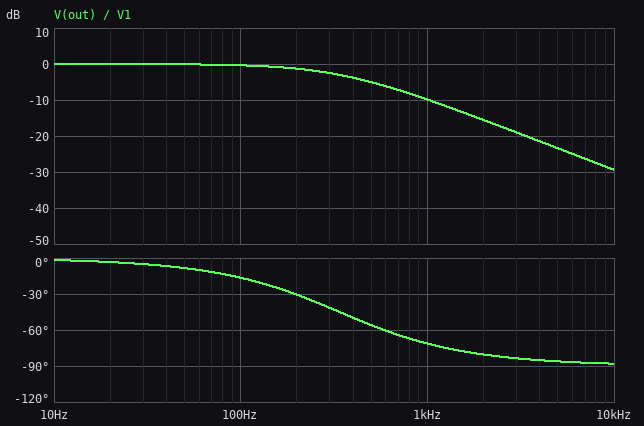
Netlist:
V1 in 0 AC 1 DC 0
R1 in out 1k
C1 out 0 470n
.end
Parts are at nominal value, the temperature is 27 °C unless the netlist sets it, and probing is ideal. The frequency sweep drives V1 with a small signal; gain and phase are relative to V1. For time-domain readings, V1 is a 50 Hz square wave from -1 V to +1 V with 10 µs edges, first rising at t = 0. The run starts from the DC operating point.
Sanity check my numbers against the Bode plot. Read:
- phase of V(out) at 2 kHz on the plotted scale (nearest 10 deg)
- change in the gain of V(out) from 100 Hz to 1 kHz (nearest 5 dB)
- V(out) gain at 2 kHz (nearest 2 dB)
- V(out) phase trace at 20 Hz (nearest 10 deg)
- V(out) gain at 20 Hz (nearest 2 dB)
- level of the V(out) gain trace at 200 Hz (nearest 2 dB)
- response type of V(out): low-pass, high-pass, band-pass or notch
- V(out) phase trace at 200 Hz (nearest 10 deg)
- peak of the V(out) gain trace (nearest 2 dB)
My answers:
-80 deg
-10 dB
-16 dB
0 deg
0 dB
-2 dB
low-pass
-30 deg
0 dB
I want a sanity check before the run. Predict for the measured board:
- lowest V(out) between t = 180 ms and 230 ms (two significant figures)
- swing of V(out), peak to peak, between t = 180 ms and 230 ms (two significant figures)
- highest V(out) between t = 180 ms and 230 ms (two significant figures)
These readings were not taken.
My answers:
-1.0 V
2.0 V
1.0 V
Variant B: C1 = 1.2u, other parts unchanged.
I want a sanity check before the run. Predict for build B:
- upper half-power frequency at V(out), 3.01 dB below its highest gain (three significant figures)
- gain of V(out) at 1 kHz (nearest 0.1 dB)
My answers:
133 Hz
-17.6 dB
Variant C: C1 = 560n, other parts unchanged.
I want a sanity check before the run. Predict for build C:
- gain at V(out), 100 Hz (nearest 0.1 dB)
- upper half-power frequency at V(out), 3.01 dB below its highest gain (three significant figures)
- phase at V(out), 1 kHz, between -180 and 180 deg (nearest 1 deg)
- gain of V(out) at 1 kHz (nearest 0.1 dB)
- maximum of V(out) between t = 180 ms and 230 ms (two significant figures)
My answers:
-0.5 dB
284 Hz
-74 deg
-11.3 dB
1.0 V
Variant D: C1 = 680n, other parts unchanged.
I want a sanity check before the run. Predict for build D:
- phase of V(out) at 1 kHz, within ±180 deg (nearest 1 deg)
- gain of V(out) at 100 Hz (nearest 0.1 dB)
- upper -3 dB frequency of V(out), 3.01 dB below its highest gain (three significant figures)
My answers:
-77 deg
-0.7 dB
234 Hz
